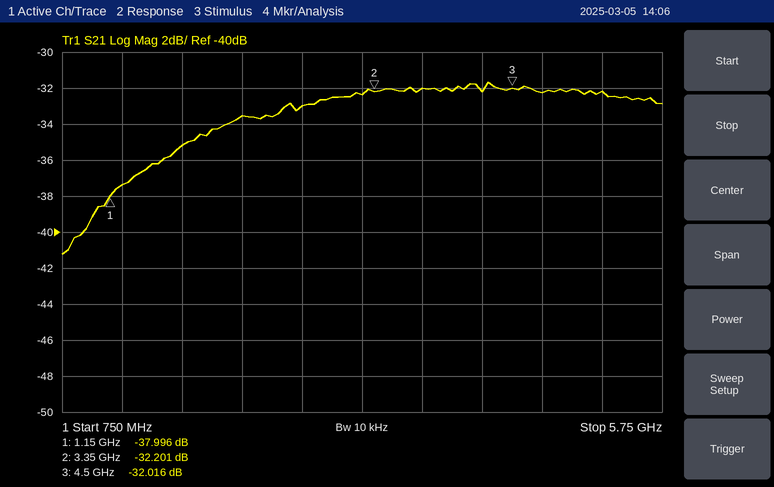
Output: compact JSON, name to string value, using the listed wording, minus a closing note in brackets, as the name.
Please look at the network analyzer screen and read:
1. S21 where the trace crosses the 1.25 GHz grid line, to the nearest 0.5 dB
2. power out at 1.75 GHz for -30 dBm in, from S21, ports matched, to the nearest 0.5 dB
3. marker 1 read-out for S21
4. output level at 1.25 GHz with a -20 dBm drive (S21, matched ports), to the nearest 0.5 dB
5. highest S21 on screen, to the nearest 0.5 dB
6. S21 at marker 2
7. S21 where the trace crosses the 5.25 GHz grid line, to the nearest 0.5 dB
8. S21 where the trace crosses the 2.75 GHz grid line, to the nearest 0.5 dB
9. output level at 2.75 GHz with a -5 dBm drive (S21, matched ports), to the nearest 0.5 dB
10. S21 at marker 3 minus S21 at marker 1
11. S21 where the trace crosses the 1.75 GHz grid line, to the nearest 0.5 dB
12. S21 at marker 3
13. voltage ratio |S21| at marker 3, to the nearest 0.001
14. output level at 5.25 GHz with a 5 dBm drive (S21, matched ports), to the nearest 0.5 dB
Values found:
{"S21 where the trace crosses the 1.25 GHz grid line, to the nearest 0.5 dB": "-37.5 dB", "power out at 1.75 GHz for -30 dBm in, from S21, ports matched, to the nearest 0.5 dB": "-65.0 dBm", "marker 1 read-out for S21": "-37.996 dB", "output level at 1.25 GHz with a -20 dBm drive (S21, matched ports), to the nearest 0.5 dB": "-57.5 dBm", "highest S21 on screen, to the nearest 0.5 dB": "-31.5 dB", "S21 at marker 2": "-32.201 dB", "S21 where the trace crosses the 5.25 GHz grid line, to the nearest 0.5 dB": "-32.0 dB", "S21 where the trace crosses the 2.75 GHz grid line, to the nearest 0.5 dB": "-33.0 dB", "output level at 2.75 GHz with a -5 dBm drive (S21, matched ports), to the nearest 0.5 dB": "-38.0 dBm", "S21 at marker 3 minus S21 at marker 1": "5.980 dB", "S21 where the trace crosses the 1.75 GHz grid line, to the nearest 0.5 dB": "-35.0 dB", "S21 at marker 3": "-32.016 dB", "voltage ratio |S21| at marker 3, to the nearest 0.001": "0.025", "output level at 5.25 GHz with a 5 dBm drive (S21, matched ports), to the nearest 0.5 dB": "-27.0 dBm"}
